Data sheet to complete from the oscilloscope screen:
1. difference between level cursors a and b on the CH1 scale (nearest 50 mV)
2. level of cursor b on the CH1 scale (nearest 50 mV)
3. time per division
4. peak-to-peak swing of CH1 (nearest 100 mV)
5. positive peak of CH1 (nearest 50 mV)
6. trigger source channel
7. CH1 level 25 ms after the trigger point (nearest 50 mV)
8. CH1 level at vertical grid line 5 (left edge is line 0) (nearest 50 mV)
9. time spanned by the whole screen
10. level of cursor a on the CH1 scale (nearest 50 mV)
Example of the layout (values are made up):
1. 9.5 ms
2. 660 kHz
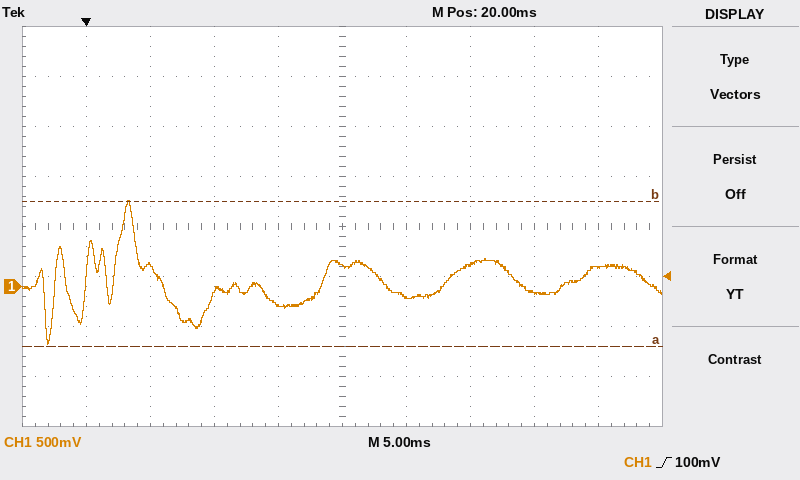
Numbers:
1. 1.45 V
2. 850 mV
3. 5 ms
4. 1.40 V
5. 850 mV
6. CH1
7. -100 mV
8. 200 mV
9. 50 ms
10. -600 mV
